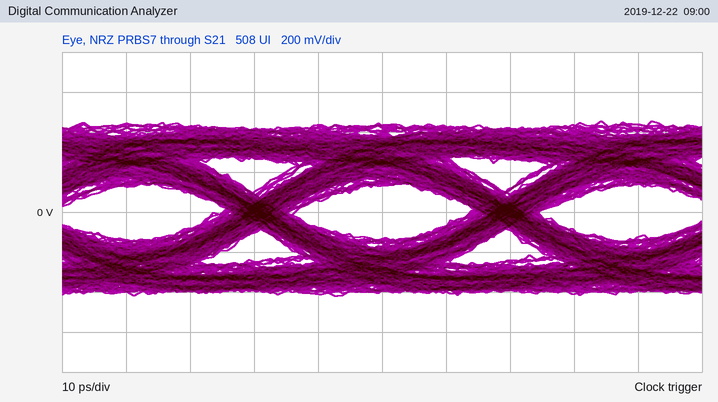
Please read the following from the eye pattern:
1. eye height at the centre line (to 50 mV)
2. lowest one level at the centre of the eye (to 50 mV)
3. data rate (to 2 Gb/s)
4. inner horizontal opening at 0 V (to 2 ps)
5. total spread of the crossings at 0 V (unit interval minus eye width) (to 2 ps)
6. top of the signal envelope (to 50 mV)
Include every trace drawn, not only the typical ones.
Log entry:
250 mV
150 mV
26 Gb/s
28 ps
12 ps
450 mV
